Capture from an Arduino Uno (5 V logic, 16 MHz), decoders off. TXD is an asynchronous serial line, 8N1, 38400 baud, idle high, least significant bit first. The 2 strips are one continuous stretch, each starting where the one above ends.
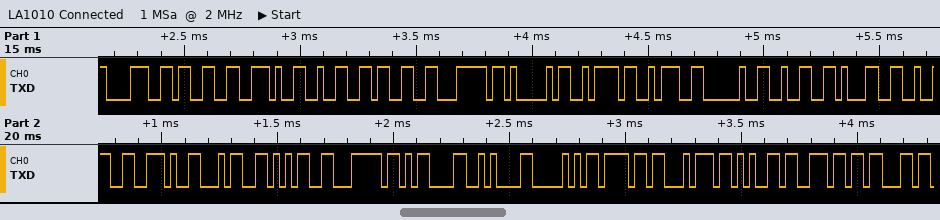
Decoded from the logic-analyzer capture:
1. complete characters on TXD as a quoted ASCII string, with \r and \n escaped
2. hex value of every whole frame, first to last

"83.23|Az: 212.45|\r\nPotenc"
38 33 2E 32 33 7C 41 7A 3A 20 32 31 32 2E 34 35 7C 0D 0A 50 6F 74 65 6E 63
